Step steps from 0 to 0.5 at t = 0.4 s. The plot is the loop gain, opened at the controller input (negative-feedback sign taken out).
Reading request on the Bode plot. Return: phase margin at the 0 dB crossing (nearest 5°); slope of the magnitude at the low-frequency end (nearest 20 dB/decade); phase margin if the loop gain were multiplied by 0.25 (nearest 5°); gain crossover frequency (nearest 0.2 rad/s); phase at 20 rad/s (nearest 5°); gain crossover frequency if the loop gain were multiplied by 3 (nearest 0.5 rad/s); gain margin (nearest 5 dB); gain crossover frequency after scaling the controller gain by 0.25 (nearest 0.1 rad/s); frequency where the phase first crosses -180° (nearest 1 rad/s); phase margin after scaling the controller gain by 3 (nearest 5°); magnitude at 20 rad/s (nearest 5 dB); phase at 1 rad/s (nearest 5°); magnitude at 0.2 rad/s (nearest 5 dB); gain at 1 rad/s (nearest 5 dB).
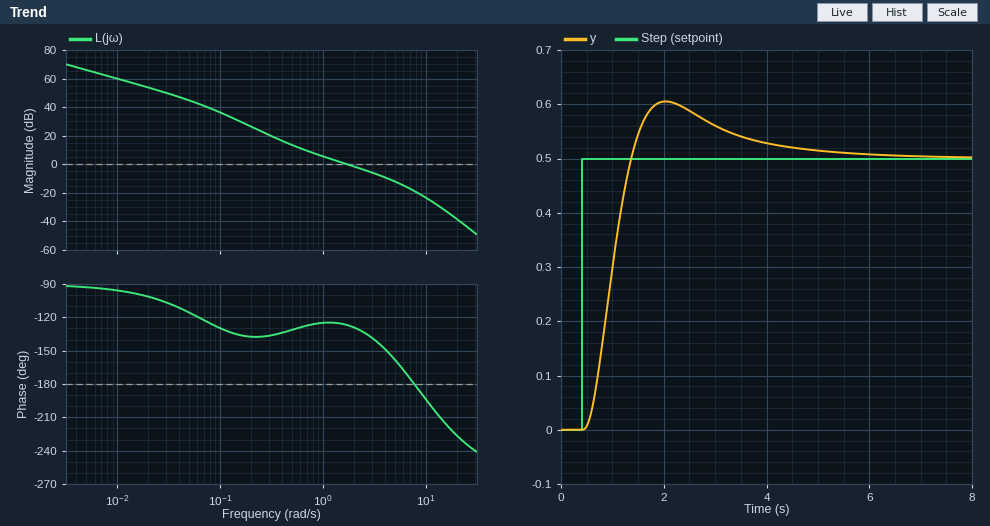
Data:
55°
-20 dB/decade
50°
1.8 rad/s
-225°
4.0 rad/s
20 dB
0.6 rad/s
8 rad/s
30°
-40 dB
-125°
25 dB
5 dB
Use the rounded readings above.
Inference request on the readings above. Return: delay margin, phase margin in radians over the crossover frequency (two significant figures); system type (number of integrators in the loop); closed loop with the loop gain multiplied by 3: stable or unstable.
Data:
0.53 s
1
stable
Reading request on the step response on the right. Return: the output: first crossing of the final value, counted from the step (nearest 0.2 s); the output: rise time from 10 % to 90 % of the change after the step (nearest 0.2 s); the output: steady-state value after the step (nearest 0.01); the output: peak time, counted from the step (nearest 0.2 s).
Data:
1.0 s
0.6 s
0.50
1.6 s
